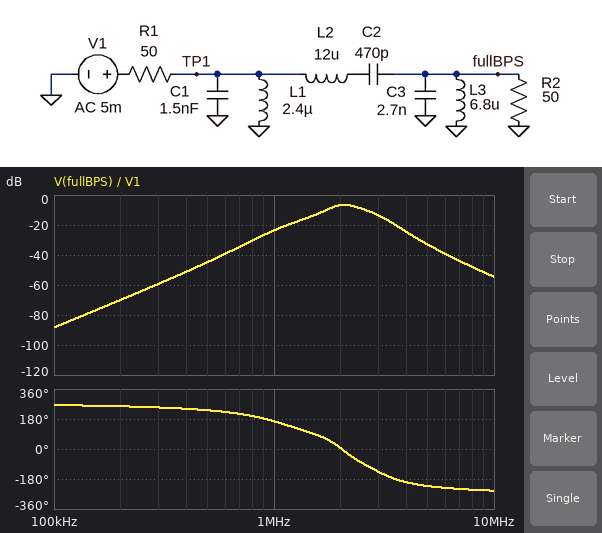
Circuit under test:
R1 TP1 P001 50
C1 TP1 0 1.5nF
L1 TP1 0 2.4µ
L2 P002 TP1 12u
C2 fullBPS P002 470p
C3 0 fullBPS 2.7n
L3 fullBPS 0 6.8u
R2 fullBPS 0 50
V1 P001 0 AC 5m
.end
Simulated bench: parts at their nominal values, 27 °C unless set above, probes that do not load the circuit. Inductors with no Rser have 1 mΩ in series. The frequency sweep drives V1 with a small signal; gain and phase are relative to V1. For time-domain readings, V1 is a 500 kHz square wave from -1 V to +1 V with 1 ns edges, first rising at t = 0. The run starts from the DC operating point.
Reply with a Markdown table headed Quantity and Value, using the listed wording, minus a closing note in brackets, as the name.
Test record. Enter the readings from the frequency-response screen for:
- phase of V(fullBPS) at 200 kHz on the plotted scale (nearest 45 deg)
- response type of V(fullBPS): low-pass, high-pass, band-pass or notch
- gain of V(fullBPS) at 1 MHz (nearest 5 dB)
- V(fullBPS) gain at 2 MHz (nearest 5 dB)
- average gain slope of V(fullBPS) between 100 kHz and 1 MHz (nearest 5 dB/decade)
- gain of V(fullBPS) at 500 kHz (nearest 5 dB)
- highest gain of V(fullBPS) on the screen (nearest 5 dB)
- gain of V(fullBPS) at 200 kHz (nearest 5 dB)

| Quantity | Value |
|---|---|
| phase of V(fullBPS) at 200 kHz on the plotted scale | 270 deg |
| response type of V(fullBPS): low-pass, high-pass, band-pass or notch | band-pass |
| gain of V(fullBPS) at 1 MHz | -25 dB |
| V(fullBPS) gain at 2 MHz | -5 dB |
| average gain slope of V(fullBPS) between 100 kHz and 1 MHz | 65 dB/decade |
| gain of V(fullBPS) at 500 kHz | -45 dB |
| highest gain of V(fullBPS) on the screen | -5 dB |
| gain of V(fullBPS) at 200 kHz | -70 dB |
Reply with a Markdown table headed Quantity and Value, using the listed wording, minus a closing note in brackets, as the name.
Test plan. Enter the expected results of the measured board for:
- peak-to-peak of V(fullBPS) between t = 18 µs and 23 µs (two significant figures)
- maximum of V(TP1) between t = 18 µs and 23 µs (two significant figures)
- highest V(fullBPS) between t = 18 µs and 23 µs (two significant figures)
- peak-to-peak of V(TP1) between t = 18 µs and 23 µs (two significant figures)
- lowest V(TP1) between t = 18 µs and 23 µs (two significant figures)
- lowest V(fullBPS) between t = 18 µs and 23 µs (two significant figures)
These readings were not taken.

| Quantity | Value |
|---|---|
| peak-to-peak of V(fullBPS) between t = 18 µs and 23 µs | 370 mV |
| maximum of V(TP1) between t = 18 µs and 23 µs | 920 mV |
| highest V(fullBPS) between t = 18 µs and 23 µs | 190 mV |
| peak-to-peak of V(TP1) between t = 18 µs and 23 µs | 1.8 V |
| lowest V(TP1) between t = 18 µs and 23 µs | -920 mV |
| lowest V(fullBPS) between t = 18 µs and 23 µs | -190 mV |
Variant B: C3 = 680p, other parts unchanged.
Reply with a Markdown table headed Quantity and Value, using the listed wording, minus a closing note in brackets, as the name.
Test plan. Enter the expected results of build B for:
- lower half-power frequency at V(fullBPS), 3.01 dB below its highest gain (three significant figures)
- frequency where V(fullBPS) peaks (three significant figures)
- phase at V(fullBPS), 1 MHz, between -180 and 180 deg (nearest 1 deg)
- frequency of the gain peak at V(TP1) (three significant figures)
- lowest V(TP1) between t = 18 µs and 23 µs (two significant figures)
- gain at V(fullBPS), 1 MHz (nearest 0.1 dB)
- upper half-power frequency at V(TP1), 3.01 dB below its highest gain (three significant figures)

| Quantity | Value |
|---|---|
| lower half-power frequency at V(fullBPS), 3.01 dB below its highest gain | 1.59 MHz |
| frequency where V(fullBPS) peaks | 1.95 MHz |
| phase at V(fullBPS), 1 MHz, between -180 and 180 deg | -164 deg |
| frequency of the gain peak at V(TP1) | 3.29 MHz |
| lowest V(TP1) between t = 18 µs and 23 µs | -950 mV |
| gain at V(fullBPS), 1 MHz | -25.5 dB |
| upper half-power frequency at V(TP1), 3.01 dB below its highest gain | 4.58 MHz |
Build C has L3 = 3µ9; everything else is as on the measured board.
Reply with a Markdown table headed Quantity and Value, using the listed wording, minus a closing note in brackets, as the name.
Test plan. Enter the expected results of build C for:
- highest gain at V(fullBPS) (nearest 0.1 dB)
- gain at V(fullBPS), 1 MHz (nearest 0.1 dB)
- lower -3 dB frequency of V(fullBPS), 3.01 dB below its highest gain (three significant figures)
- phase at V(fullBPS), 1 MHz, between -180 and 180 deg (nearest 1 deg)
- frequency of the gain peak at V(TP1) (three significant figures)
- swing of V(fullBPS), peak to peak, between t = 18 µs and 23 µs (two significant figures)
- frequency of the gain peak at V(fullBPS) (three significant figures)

| Quantity | Value |
|---|---|
| highest gain at V(fullBPS) | -6.1 dB |
| gain at V(fullBPS), 1 MHz | -26.5 dB |
| lower -3 dB frequency of V(fullBPS), 3.01 dB below its highest gain | 1.69 MHz |
| phase at V(fullBPS), 1 MHz, between -180 and 180 deg | -156 deg |
| frequency of the gain peak at V(TP1) | 3.23 MHz |
| swing of V(fullBPS), peak to peak, between t = 18 µs and 23 µs | 410 mV |
| frequency of the gain peak at V(fullBPS) | 2.11 MHz |
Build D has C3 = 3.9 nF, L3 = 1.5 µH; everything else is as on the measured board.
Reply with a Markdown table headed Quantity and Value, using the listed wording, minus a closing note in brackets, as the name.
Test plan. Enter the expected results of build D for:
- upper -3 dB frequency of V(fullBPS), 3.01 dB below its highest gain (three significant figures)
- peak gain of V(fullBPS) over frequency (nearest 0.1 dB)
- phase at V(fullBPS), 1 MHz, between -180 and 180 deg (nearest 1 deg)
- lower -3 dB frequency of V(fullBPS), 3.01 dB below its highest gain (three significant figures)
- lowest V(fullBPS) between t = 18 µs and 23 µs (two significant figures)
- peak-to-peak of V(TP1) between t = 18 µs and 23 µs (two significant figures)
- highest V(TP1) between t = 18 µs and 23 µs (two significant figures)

| Quantity | Value |
|---|---|
| upper -3 dB frequency of V(fullBPS), 3.01 dB below its highest gain | 2.70 MHz |
| peak gain of V(fullBPS) over frequency | -6.1 dB |
| phase at V(fullBPS), 1 MHz, between -180 and 180 deg | -125 deg |
| lower -3 dB frequency of V(fullBPS), 3.01 dB below its highest gain | 1.62 MHz |
| lowest V(fullBPS) between t = 18 µs and 23 µs | -180 mV |
| peak-to-peak of V(TP1) between t = 18 µs and 23 µs | 1.9 V |
| highest V(TP1) between t = 18 µs and 23 µs | 950 mV |
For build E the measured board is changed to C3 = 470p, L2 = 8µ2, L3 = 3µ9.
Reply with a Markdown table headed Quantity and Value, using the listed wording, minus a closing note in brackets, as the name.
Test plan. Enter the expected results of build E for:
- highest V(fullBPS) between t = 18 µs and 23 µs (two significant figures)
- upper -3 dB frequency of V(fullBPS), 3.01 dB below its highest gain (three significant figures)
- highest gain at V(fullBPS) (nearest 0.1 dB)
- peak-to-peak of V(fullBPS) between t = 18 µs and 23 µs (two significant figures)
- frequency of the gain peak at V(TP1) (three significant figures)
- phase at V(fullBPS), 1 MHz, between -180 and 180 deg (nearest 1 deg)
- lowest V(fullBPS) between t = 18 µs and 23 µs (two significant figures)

| Quantity | Value |
|---|---|
| highest V(fullBPS) between t = 18 µs and 23 µs | 270 mV |
| upper -3 dB frequency of V(fullBPS), 3.01 dB below its highest gain | 3.69 MHz |
| highest gain at V(fullBPS) | -6.0 dB |
| peak-to-peak of V(fullBPS) between t = 18 µs and 23 µs | 530 mV |
| frequency of the gain peak at V(TP1) | 3.57 MHz |
| phase at V(fullBPS), 1 MHz, between -180 and 180 deg | -141 deg |
| lowest V(fullBPS) between t = 18 µs and 23 µs | -270 mV |
